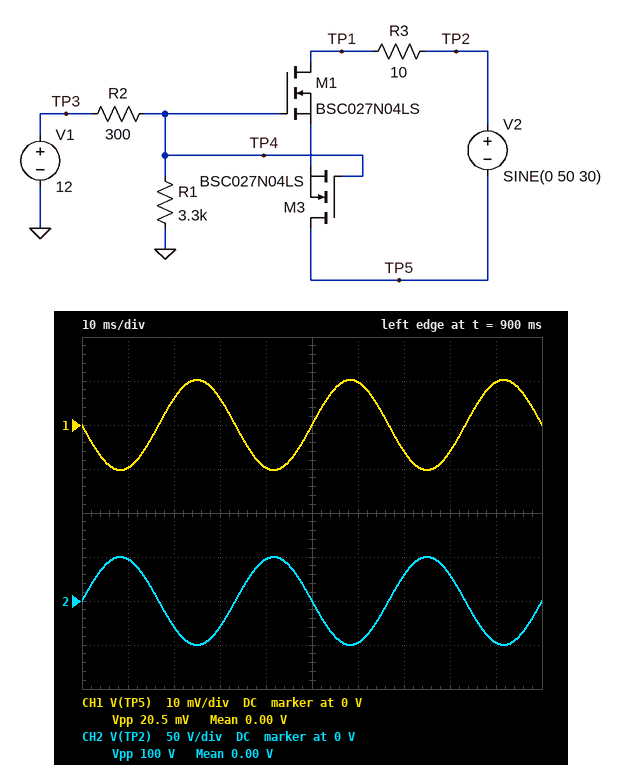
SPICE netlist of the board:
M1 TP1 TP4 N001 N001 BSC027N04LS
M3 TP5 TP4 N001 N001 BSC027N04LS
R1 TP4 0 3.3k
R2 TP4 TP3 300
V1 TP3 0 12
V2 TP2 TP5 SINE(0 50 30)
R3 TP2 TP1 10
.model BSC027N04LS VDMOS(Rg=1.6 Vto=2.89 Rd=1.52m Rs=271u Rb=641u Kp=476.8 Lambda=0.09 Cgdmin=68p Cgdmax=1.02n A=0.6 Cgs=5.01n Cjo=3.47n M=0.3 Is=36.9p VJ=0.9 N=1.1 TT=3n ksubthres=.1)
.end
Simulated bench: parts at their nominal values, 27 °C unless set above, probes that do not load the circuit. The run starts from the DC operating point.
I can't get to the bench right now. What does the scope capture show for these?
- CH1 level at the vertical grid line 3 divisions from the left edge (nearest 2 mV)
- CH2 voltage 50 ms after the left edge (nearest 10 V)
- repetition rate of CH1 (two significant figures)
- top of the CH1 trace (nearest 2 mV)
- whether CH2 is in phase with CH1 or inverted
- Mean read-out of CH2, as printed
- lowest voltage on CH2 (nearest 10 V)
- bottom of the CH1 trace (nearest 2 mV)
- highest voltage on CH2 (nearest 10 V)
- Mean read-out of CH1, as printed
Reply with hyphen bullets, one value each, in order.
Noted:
- 6 mV
- 0 V
- 30 Hz
- 10 mV
- inverted
- 0.00 V
- -50 V
- -10 mV
- 50 V
- 0.00 V
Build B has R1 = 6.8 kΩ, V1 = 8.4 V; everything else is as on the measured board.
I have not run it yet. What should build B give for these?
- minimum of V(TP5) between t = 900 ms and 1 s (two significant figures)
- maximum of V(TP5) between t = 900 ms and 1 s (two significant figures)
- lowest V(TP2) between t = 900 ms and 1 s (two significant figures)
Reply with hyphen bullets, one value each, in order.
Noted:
- -11 mV
- 11 mV
- -50 V
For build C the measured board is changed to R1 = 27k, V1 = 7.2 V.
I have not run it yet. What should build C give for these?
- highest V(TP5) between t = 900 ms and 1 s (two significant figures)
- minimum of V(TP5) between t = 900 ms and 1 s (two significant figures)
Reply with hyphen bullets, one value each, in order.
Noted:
- 11 mV
- -11 mV
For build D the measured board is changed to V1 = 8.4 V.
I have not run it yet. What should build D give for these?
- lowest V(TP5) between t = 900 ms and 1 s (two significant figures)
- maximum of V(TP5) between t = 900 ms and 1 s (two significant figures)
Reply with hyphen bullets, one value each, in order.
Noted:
- -11 mV
- 11 mV
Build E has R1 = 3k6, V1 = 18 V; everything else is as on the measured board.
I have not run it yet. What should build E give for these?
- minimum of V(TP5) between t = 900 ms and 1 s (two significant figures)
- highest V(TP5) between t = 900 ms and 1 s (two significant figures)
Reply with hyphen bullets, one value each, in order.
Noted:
- -9.7 mV
- 9.7 mV
